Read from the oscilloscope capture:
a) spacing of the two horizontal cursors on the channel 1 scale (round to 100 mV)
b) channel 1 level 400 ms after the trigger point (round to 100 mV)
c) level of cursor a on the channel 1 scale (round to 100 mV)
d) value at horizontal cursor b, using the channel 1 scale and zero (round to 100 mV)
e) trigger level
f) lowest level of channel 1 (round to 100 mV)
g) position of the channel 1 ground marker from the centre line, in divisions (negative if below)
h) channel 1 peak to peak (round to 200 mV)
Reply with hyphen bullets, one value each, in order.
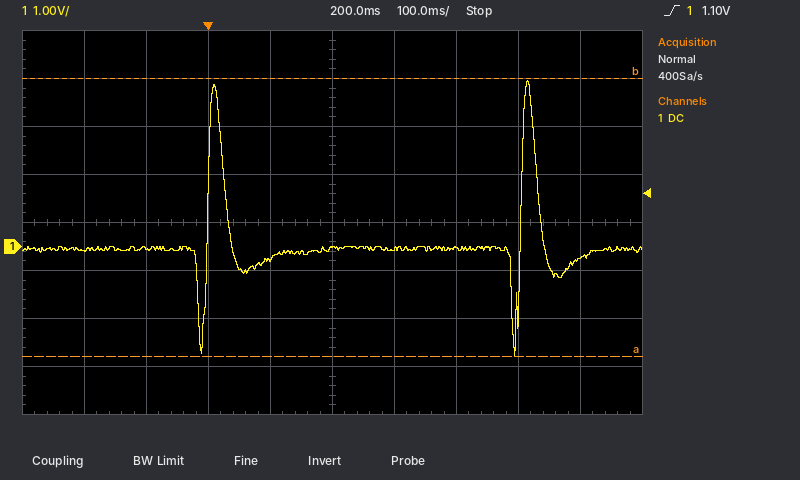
- 5.8 V
- 0.0 V
- -2.3 V
- 3.5 V
- 1.10 V
- -2.3 V
- -0.5 div
- 5.8 V
